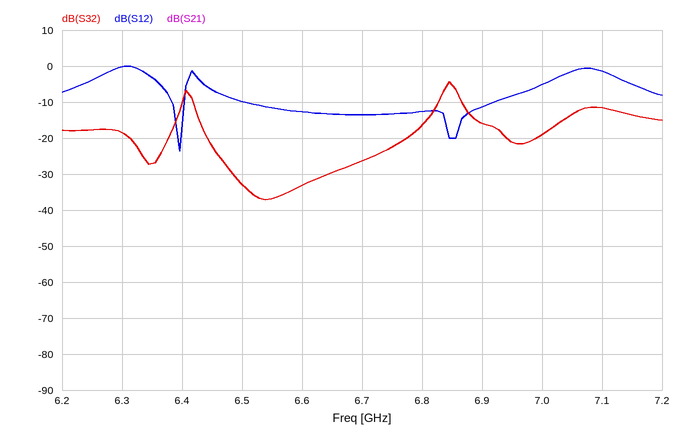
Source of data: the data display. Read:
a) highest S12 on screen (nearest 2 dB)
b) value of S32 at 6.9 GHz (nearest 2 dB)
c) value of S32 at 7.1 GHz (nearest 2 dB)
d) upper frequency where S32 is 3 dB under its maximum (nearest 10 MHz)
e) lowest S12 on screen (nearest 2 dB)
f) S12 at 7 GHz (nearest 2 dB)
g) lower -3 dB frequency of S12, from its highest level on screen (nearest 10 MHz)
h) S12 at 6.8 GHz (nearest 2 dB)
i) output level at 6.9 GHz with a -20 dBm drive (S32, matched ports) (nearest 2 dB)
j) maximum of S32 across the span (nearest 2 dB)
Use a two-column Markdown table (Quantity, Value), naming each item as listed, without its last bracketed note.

| Quantity | Value |
|---|---|
| highest S12 on screen | 0 dB |
| value of S32 at 6.9 GHz | -16 dB |
| value of S32 at 7.1 GHz | -12 dB |
| upper frequency where S32 is 3 dB under its maximum | 6.86 GHz |
| lowest S12 on screen | -24 dB |
| S12 at 7 GHz | -6 dB |
| lower -3 dB frequency of S12, from its highest level on screen | 6.26 GHz |
| S12 at 6.8 GHz | -12 dB |
| output level at 6.9 GHz with a -20 dBm drive (S32, matched ports) | -36 dBm |
| maximum of S32 across the span | -4 dB |
